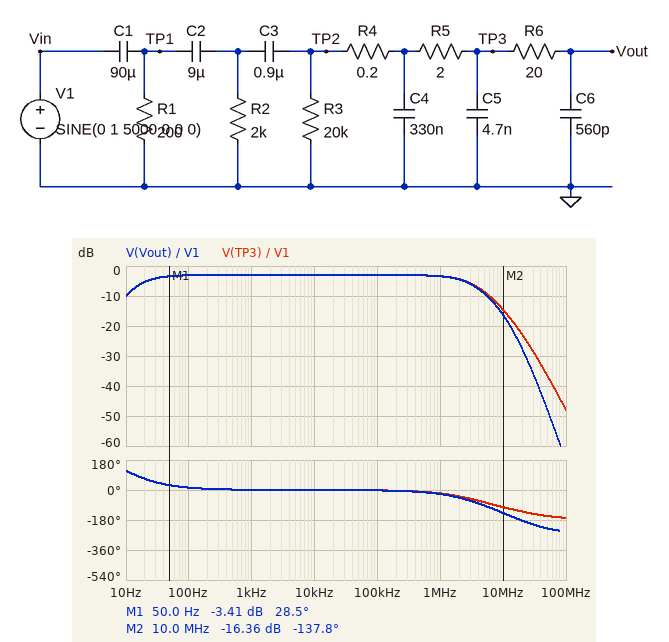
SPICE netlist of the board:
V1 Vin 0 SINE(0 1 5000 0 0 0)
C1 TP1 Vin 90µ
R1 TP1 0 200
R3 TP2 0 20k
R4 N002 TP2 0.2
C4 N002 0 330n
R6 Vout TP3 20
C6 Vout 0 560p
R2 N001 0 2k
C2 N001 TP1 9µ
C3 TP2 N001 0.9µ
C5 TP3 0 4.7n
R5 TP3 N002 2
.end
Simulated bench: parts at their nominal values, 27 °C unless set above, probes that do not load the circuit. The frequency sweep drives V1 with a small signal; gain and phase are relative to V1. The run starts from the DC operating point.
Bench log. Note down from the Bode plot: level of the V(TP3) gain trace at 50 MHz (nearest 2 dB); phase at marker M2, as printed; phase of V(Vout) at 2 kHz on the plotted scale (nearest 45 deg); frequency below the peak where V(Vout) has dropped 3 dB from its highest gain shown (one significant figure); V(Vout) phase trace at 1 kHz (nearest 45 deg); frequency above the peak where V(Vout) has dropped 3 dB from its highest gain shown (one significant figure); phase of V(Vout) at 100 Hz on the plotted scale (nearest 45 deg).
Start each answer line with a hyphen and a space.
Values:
- -36 dB
- -137.8 deg
- 0 deg
- 20 Hz
- 0 deg
- 3 MHz
- 0 deg
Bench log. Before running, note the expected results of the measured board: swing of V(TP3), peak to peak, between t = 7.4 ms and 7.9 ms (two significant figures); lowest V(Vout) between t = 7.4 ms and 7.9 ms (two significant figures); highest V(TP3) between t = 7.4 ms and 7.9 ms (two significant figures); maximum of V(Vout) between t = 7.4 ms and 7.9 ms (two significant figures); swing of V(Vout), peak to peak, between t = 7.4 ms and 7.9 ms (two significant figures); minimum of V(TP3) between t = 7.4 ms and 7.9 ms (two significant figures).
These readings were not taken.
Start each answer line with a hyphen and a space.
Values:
- 1.4 V
- -710 mV
- 710 mV
- 710 mV
- 1.4 V
- -710 mV
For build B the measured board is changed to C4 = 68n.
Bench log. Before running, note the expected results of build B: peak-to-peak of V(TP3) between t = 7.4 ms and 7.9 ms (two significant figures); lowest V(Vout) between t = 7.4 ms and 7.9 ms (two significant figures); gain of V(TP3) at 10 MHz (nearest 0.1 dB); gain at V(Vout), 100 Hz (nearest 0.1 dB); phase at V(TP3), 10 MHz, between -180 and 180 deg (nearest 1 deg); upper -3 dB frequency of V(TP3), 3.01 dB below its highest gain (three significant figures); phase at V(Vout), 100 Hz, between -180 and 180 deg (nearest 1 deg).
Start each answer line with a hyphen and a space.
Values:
- 1.8 V
- -920 mV
- -4.8 dB
- -0.9 dB
- -70 deg
- 8.24 MHz
- 16 deg
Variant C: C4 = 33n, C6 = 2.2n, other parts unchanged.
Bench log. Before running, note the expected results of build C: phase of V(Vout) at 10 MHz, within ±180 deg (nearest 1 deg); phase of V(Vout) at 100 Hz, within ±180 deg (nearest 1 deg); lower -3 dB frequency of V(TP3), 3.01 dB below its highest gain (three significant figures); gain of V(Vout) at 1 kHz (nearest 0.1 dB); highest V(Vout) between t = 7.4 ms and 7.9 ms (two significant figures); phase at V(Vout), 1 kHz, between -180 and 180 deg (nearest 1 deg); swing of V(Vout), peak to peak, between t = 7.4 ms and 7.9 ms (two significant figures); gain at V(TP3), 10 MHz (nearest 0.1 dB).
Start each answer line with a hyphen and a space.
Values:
- -123 deg
- 16 deg
- 18.9 Hz
- -0.4 dB
- 950 mV
- 2 deg
- 1.9 V
- -3.3 dB
